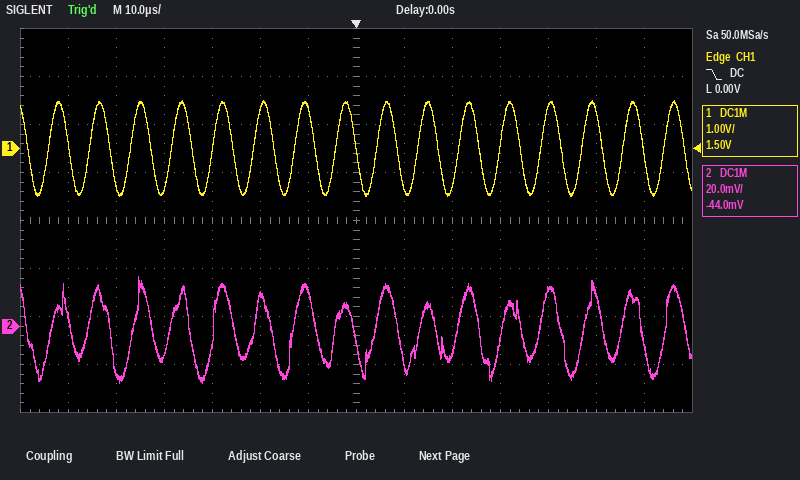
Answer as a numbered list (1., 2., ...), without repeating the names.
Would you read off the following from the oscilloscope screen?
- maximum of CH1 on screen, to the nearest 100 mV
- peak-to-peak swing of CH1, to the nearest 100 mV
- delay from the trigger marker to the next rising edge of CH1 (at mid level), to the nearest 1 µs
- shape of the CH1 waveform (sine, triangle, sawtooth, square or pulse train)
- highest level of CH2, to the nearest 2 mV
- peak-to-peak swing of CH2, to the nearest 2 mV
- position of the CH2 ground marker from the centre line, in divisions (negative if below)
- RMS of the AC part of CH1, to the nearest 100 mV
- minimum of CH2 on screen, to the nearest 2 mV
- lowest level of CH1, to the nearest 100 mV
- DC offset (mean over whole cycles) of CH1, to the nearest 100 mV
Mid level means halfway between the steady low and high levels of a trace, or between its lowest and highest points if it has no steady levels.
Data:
1. 1.0 V
2. 2.0 V
3. 4 µs
4. sine
5. 20 mV
6. 44 mV
7. -2.2 div
8. 700 mV
9. -24 mV
10. -1.0 V
11. 0.0 V
